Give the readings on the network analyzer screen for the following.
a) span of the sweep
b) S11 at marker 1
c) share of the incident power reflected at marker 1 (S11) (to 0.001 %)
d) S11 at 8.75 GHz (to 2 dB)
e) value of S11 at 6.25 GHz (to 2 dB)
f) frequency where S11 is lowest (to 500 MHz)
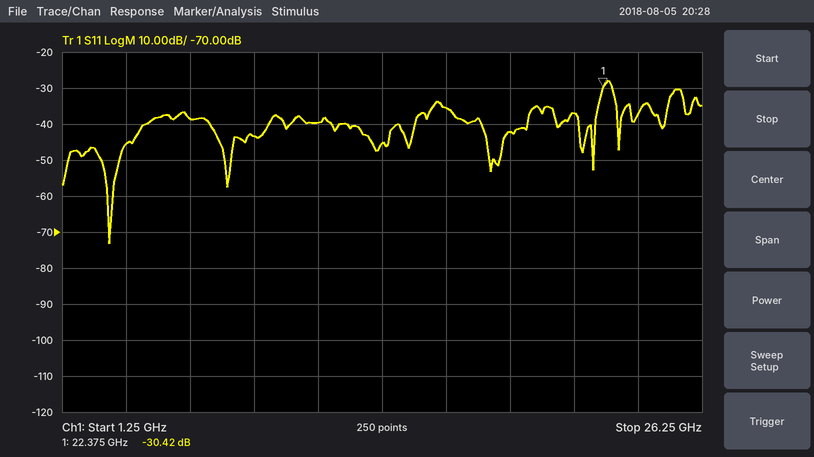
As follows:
25 GHz
-30.42 dB
0.091 %
-44 dB
-38 dB
3.0 GHz
